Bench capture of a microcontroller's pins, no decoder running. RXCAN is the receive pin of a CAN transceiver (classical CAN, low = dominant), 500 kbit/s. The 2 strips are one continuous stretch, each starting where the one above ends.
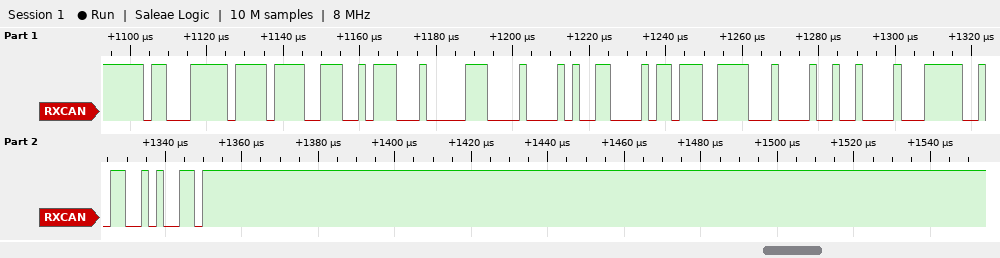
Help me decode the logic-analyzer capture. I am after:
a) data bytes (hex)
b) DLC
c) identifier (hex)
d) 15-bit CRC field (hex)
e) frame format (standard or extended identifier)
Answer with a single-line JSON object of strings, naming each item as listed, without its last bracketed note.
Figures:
{"data bytes": "30 85 30 B7 3C 42 48 47", "DLC": "8", "identifier": "0x18FEF397", "15-bit CRC field": "0x6B29", "frame format": "extended"}
